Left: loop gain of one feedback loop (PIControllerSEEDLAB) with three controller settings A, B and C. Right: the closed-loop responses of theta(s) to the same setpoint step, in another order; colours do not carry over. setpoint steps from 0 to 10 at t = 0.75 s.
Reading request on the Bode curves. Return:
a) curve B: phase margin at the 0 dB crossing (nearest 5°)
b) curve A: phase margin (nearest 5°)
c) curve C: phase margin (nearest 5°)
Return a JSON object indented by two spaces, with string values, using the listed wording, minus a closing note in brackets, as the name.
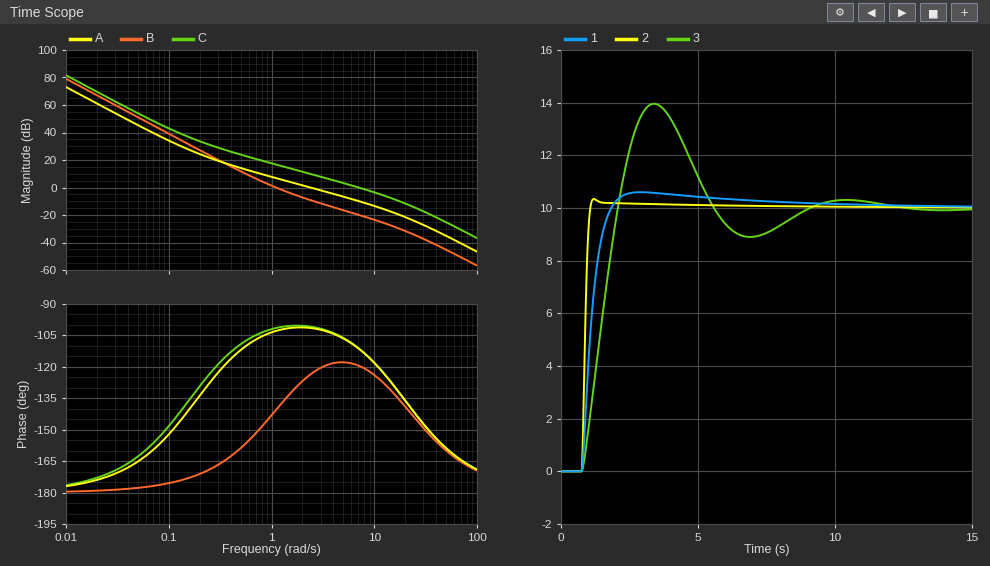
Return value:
{
  "curve B: phase margin at the 0 dB crossing": "40°",
  "curve A: phase margin": "80°",
  "curve C: phase margin": "70°"
}
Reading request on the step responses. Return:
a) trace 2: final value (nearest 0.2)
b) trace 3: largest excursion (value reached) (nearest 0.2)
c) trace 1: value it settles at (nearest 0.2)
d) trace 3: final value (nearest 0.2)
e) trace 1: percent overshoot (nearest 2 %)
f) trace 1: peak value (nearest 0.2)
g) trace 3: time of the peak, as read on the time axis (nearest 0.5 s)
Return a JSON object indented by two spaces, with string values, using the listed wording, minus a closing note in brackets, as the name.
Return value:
{
  "trace 2: final value": "10.0",
  "trace 3: largest excursion (value reached)": "14.0",
  "trace 1: value it settles at": "10.0",
  "trace 3: final value": "10.0",
  "trace 1: percent overshoot": "6 %",
  "trace 1: peak value": "10.6",
  "trace 3: time of the peak, as read on the time axis": "3.5 s"
}
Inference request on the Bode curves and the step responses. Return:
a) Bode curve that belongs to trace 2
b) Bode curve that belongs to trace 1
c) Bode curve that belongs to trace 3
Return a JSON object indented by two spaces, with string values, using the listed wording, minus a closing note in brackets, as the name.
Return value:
{
  "Bode curve that belongs to trace 2": "C",
  "Bode curve that belongs to trace 1": "A",
  "Bode curve that belongs to trace 3": "B"
}
